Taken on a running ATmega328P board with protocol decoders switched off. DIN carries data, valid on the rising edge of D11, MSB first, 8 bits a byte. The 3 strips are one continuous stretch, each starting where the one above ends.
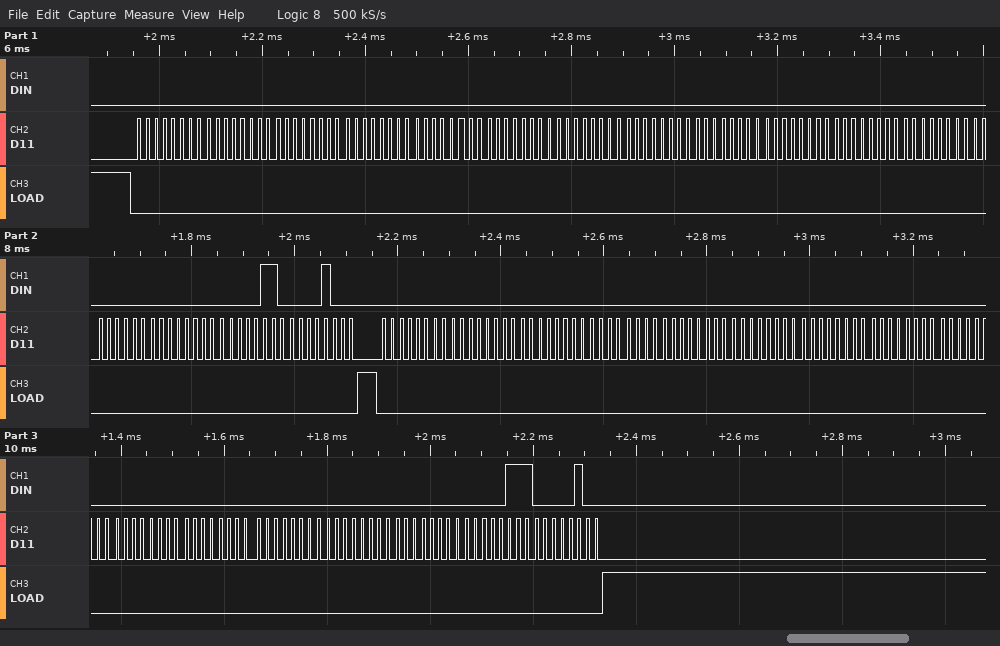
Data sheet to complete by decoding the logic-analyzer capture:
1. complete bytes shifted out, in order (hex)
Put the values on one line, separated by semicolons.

00 00 00 00 00 00 00 00 00 00 00 00 00 00 06 08 00 00 00 00 00 00 00 00 00 00 00 00 00 00 07 04
